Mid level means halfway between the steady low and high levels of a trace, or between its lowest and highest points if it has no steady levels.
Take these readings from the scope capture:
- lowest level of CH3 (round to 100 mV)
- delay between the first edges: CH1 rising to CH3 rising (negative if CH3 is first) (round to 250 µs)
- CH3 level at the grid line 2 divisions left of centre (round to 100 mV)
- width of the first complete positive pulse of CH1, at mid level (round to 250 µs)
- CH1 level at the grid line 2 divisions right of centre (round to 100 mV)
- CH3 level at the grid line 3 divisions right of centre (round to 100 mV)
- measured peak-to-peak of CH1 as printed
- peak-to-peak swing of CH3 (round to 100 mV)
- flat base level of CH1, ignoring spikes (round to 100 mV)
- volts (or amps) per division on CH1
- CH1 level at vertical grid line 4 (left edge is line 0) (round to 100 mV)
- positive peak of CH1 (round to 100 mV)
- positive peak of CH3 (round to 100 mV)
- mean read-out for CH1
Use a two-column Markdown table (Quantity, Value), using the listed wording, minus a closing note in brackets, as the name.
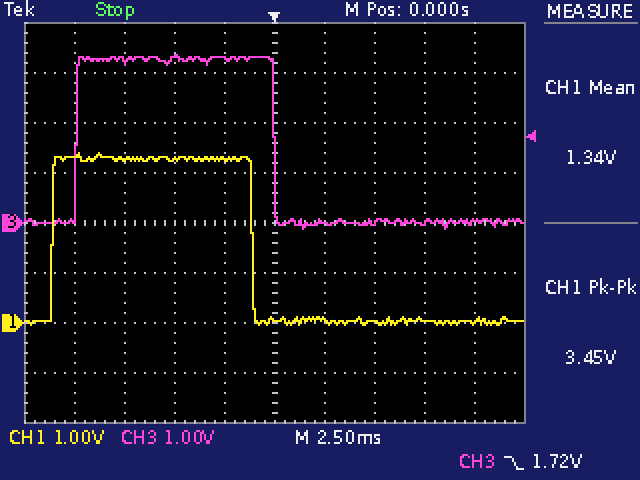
| Quantity | Value |
|---|---|
| lowest level of CH3 | -100 mV |
| delay between the first edges: CH1 rising to CH3 rising (negative if CH3 is first) | +1.25 ms |
| CH3 level at the grid line 2 divisions left of centre | 3.3 V |
| width of the first complete positive pulse of CH1, at mid level | 10.00 ms |
| CH1 level at the grid line 2 divisions right of centre | 0.0 V |
| CH3 level at the grid line 3 divisions right of centre | 0.0 V |
| measured peak-to-peak of CH1 as printed | 3.45 V |
| peak-to-peak swing of CH3 | 3.5 V |
| flat base level of CH1, ignoring spikes | 0.0 V |
| volts (or amps) per division on CH1 | 1 V |
| CH1 level at vertical grid line 4 (left edge is line 0) | 3.3 V |
| positive peak of CH1 | 3.4 V |
| positive peak of CH3 | 3.4 V |
| mean read-out for CH1 | 1.34 V |
